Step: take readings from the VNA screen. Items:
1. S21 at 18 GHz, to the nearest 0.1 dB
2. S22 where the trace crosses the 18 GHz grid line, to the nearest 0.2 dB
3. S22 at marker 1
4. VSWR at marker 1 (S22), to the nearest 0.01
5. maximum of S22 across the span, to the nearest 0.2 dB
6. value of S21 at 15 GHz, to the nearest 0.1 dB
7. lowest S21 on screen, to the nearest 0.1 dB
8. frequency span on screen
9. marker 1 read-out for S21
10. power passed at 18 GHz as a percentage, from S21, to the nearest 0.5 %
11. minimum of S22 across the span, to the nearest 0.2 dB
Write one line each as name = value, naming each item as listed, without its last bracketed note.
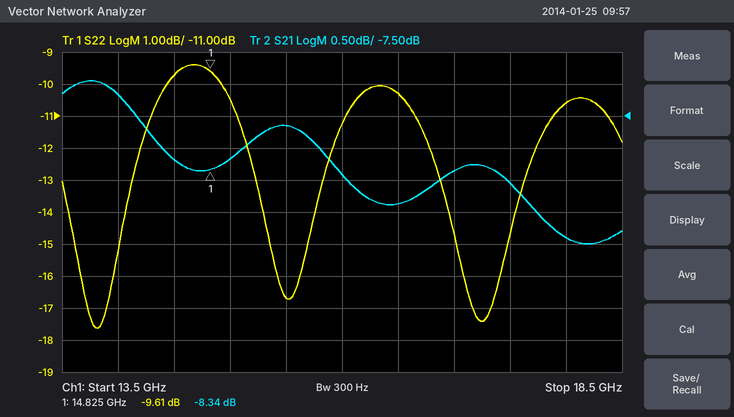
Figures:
S21 at 18 GHz, to the nearest 0.1 dB = -9.4 dB
S22 where the trace crosses the 18 GHz grid line, to the nearest 0.2 dB = -10.6 dB
S22 at marker 1 = -9.61 dB
VSWR at marker 1 (S22), to the nearest 0.01 = 1.99
maximum of S22 across the span, to the nearest 0.2 dB = -9.4 dB
value of S21 at 15 GHz, to the nearest 0.1 dB = -8.2 dB
lowest S21 on screen, to the nearest 0.1 dB = -9.5 dB
frequency span on screen = 5 GHz
marker 1 read-out for S21 = -8.34 dB
power passed at 18 GHz as a percentage, from S21, to the nearest 0.5 % = 11.5 %
minimum of S22 across the span, to the nearest 0.2 dB = -17.6 dB
